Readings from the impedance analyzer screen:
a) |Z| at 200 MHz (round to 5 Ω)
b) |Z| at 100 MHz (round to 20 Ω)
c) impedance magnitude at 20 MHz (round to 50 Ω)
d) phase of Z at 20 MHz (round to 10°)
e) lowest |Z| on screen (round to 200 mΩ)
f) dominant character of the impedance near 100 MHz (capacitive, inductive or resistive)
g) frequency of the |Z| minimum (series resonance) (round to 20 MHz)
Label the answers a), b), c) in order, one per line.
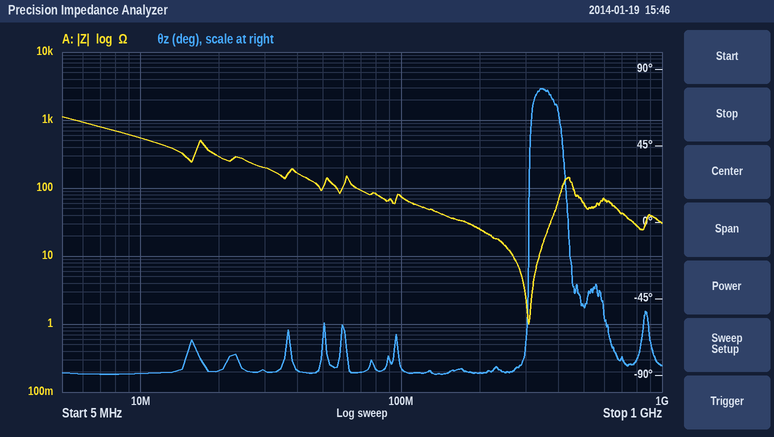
a) 25 Ω
b) 80 Ω
c) 300 Ω
d) -90°
e) 1.0 Ω
f) capacitive
g) 300 MHz
